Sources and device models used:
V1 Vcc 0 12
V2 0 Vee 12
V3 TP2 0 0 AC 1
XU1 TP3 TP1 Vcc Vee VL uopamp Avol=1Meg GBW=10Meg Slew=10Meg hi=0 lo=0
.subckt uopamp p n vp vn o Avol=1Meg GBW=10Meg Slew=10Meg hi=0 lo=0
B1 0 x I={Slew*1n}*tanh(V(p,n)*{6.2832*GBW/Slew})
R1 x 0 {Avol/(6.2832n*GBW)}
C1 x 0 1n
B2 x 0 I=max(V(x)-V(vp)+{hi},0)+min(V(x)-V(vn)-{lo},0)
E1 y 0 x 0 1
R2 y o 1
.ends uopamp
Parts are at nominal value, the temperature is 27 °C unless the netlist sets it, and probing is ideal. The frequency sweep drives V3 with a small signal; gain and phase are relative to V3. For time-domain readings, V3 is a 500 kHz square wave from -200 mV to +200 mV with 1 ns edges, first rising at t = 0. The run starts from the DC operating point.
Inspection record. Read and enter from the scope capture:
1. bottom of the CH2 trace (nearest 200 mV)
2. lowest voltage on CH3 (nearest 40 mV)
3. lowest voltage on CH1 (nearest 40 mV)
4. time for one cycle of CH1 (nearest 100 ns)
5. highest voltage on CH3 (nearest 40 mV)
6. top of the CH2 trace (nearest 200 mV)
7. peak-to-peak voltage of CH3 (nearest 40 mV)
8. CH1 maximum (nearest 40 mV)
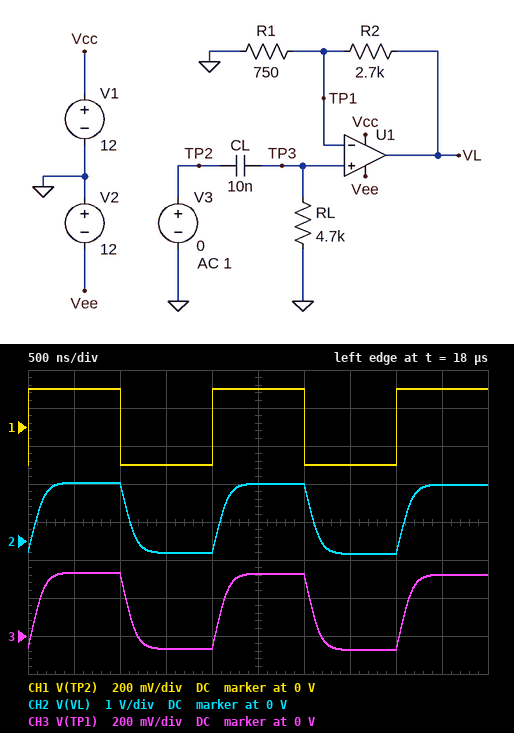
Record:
-400 mV
-80 mV
-200 mV
2.0 µs
320 mV
1.6 V
400 mV
200 mV
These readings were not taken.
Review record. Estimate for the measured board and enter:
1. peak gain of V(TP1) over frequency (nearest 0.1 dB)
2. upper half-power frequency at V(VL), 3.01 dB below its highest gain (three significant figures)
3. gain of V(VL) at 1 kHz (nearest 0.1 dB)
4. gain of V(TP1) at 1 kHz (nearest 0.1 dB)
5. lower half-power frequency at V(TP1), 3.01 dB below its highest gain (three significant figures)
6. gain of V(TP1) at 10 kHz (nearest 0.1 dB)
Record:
0 dB
2.18 MHz
2.3 dB
-11.0 dB
3.38 kHz
-0.5 dB
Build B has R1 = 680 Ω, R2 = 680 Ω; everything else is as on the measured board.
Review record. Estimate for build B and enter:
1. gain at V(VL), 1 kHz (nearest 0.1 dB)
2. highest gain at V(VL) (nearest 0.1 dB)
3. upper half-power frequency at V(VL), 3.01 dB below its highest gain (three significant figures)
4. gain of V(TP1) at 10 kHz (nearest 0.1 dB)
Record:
-4.9 dB
6.0 dB
5.00 MHz
-0.5 dB
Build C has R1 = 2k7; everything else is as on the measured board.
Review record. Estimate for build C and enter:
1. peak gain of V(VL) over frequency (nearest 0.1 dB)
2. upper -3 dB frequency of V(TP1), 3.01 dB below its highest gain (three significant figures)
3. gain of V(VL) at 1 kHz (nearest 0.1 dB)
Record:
6.0 dB
5.01 MHz
-4.9 dB
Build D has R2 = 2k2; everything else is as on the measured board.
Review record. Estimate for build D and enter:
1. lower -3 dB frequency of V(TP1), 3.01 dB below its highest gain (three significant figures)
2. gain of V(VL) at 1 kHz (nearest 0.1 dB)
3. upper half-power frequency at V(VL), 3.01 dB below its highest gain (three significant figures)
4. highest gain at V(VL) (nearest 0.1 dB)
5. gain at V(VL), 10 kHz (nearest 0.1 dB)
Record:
3.38 kHz
0.9 dB
2.55 MHz
11.9 dB
11.4 dB
